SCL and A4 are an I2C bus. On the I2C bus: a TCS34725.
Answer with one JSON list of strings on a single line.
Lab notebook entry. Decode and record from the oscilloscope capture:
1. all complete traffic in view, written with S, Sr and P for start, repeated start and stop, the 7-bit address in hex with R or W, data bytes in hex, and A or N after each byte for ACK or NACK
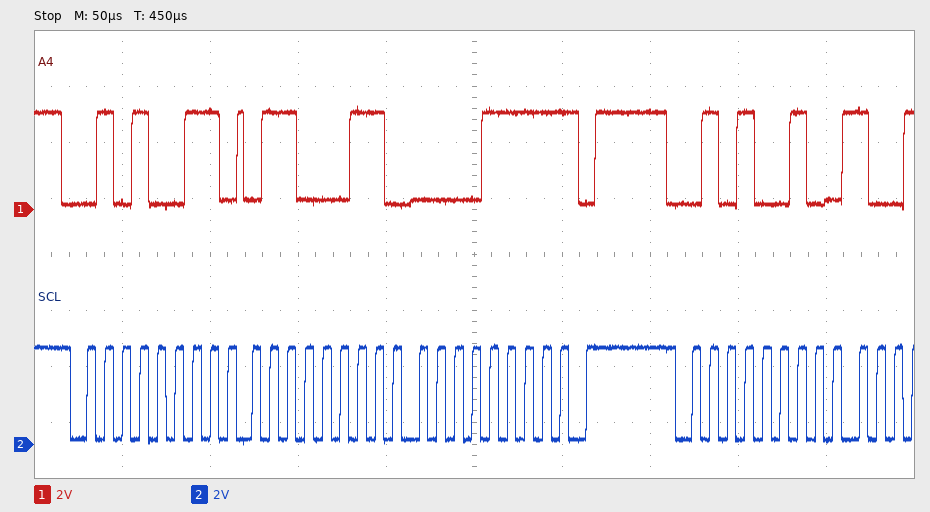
["S 29R A 63 A 0F N P S 29W A"]
